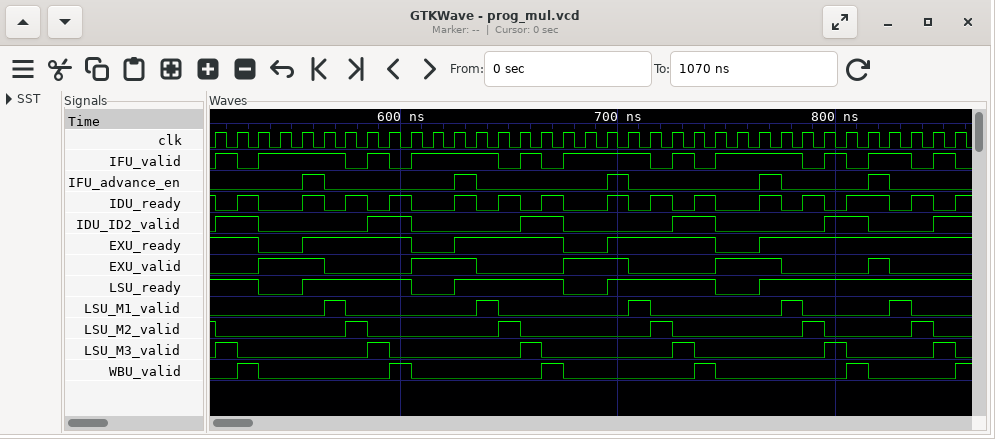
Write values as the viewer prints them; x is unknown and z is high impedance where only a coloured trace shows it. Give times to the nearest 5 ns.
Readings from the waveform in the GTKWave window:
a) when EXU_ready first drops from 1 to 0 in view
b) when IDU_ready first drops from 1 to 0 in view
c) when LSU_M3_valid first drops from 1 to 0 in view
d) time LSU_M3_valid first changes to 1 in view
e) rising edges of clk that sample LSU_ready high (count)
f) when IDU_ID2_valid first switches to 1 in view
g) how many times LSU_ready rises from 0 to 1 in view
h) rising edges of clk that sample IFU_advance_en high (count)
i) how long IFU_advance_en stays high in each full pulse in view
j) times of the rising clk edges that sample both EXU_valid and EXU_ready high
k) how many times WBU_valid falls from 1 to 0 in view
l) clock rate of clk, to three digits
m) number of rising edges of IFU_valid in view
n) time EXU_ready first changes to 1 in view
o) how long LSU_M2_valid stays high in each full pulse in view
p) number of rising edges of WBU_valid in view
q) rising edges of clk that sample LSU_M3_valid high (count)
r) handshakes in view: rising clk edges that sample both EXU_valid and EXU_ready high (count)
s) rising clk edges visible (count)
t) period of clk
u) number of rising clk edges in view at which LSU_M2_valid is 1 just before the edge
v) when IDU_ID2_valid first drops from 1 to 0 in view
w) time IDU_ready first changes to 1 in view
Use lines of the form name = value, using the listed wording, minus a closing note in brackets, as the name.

when EXU_ready first drops from 1 to 0 in view = 535 ns
when IDU_ready first drops from 1 to 0 in view = 515 ns
when LSU_M3_valid first drops from 1 to 0 in view = 525 ns
time LSU_M3_valid first changes to 1 in view = 515 ns
rising edges of clk that sample LSU_ready high = 27
when IDU_ID2_valid first switches to 1 in view = 515 ns
how many times LSU_ready rises from 0 to 1 in view = 4
rising edges of clk that sample IFU_advance_en high = 5
how long IFU_advance_en stays high in each full pulse in view = 10 ns, 10 ns, 10 ns, 10 ns, 10 ns
times of the rising clk edges that sample both EXU_valid and EXU_ready high = 565 ns, 635 ns, 705 ns, 775 ns, 825 ns
how many times WBU_valid falls from 1 to 0 in view = 5
clock rate of clk, to three digits = 100 MHz
number of rising edges of IFU_valid in view = 11
time EXU_ready first changes to 1 in view = 555 ns
how long LSU_M2_valid stays high in each full pulse in view = 10 ns, 10 ns, 10 ns, 10 ns, 10 ns
number of rising edges of WBU_valid in view = 6
rising edges of clk that sample LSU_M3_valid high = 6
handshakes in view: rising clk edges that sample both EXU_valid and EXU_ready high = 5
rising clk edges visible = 35
period of clk = 10 ns
number of rising clk edges in view at which LSU_M2_valid is 1 just before the edge = 6
when IDU_ID2_valid first drops from 1 to 0 in view = 535 ns
time IDU_ready first changes to 1 in view = 525 ns
